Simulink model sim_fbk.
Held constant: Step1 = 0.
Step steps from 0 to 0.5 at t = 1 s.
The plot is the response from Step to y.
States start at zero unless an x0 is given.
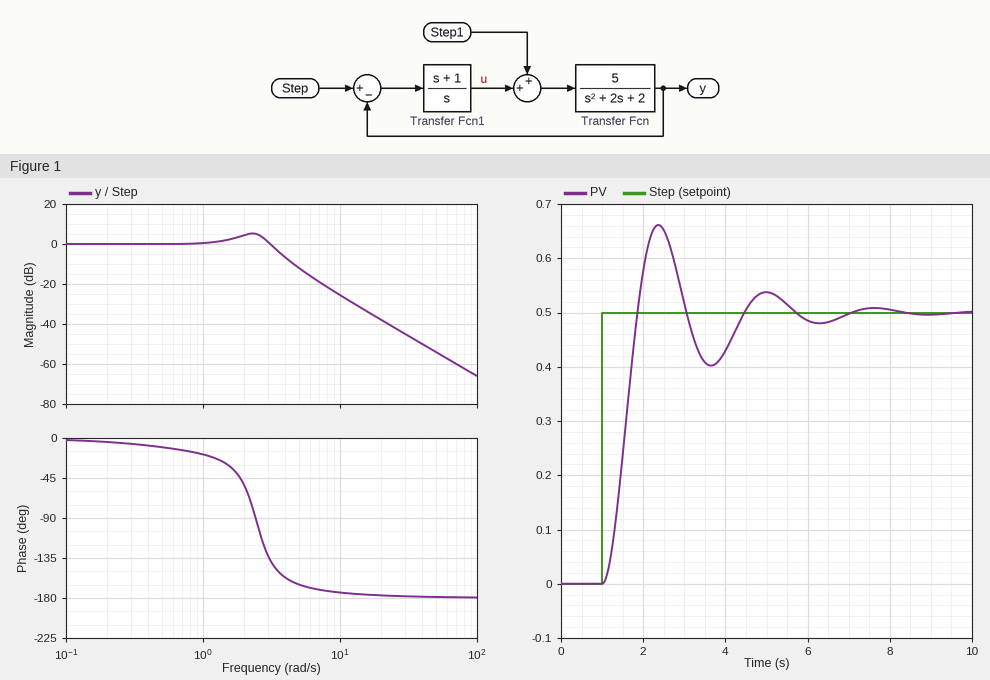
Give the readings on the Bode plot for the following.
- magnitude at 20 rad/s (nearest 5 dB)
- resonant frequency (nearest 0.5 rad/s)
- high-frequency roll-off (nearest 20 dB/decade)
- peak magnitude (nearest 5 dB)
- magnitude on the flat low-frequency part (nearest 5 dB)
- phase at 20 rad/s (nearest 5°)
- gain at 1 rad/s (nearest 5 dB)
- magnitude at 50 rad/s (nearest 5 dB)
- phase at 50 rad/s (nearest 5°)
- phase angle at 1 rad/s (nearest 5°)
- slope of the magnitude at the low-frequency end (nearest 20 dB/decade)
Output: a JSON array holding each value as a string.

["-40 dB", "2.5 rad/s", "-40 dB/decade", "5 dB", "0 dB", "-175°", "0 dB", "-55 dB", "-180°", "-20°", "0 dB/decade"]
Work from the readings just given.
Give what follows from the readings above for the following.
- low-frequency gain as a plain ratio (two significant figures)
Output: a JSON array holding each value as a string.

["1.0"]
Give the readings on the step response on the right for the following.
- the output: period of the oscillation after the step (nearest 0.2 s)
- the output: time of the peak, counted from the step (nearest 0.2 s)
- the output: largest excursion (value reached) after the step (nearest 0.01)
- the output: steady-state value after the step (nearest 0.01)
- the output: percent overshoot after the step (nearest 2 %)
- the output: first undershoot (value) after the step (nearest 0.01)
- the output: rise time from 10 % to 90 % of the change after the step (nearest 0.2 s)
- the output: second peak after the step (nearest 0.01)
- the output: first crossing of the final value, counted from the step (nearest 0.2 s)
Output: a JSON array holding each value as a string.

["2.6 s", "1.4 s", "0.66", "0.50", "32 %", "0.40", "0.6 s", "0.54", "0.8 s"]
